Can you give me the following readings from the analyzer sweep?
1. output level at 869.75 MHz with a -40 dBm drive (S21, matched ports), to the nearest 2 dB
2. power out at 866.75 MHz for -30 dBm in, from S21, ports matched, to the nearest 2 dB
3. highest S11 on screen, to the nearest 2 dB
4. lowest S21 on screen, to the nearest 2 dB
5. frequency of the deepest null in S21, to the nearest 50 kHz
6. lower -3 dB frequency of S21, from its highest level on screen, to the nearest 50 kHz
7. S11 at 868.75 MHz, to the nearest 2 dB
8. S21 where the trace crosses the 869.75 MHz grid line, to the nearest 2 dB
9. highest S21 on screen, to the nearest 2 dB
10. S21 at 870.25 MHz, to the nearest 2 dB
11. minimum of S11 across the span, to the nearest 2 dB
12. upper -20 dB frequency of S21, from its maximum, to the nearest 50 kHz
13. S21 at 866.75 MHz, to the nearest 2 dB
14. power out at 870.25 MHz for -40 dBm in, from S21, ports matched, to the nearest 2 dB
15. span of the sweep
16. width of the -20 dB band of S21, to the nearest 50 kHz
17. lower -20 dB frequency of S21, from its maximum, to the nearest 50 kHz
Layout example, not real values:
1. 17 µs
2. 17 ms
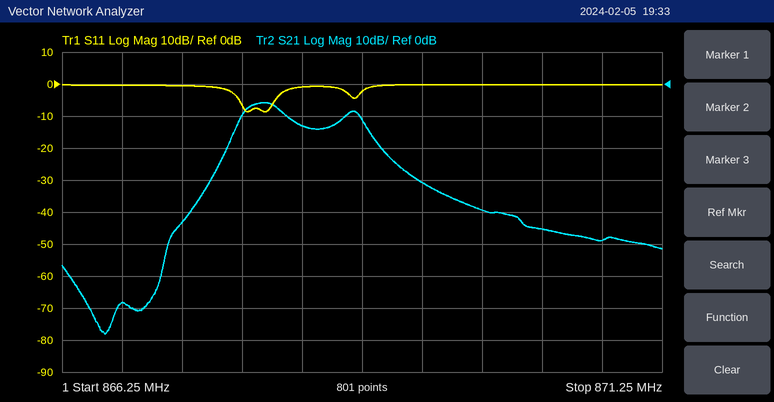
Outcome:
1. -80 dBm
2. -98 dBm
3. 0 dB
4. -78 dB
5. 866.60 MHz
6. 867.75 MHz
7. -2 dB
8. -40 dB
9. -6 dB
10. -46 dB
11. -8 dB
12. 869.05 MHz
13. -68 dB
14. -86 dBm
15. 5 MHz
16. 1.50 MHz
17. 867.55 MHz
